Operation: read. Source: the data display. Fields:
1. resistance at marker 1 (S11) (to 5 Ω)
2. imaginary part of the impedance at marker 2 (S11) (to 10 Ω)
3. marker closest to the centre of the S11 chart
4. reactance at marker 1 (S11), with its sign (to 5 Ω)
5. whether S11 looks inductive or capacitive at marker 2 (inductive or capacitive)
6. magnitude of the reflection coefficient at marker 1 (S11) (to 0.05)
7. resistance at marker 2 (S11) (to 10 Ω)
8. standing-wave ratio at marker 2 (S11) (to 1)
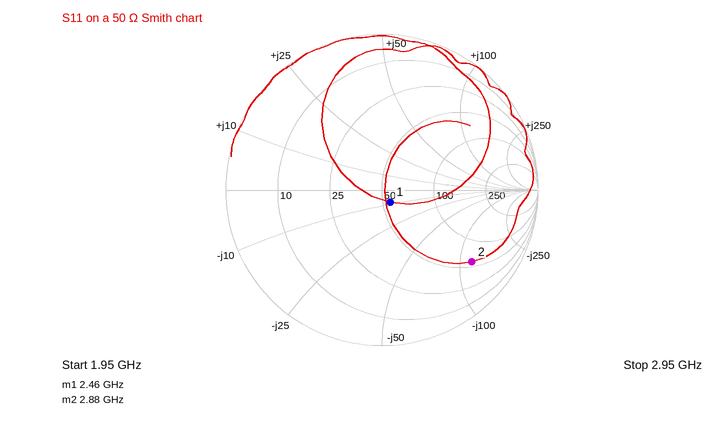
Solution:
55 Ω
-120 Ω
marker 1
-10 Ω
capacitive
0.10
60 Ω
7
